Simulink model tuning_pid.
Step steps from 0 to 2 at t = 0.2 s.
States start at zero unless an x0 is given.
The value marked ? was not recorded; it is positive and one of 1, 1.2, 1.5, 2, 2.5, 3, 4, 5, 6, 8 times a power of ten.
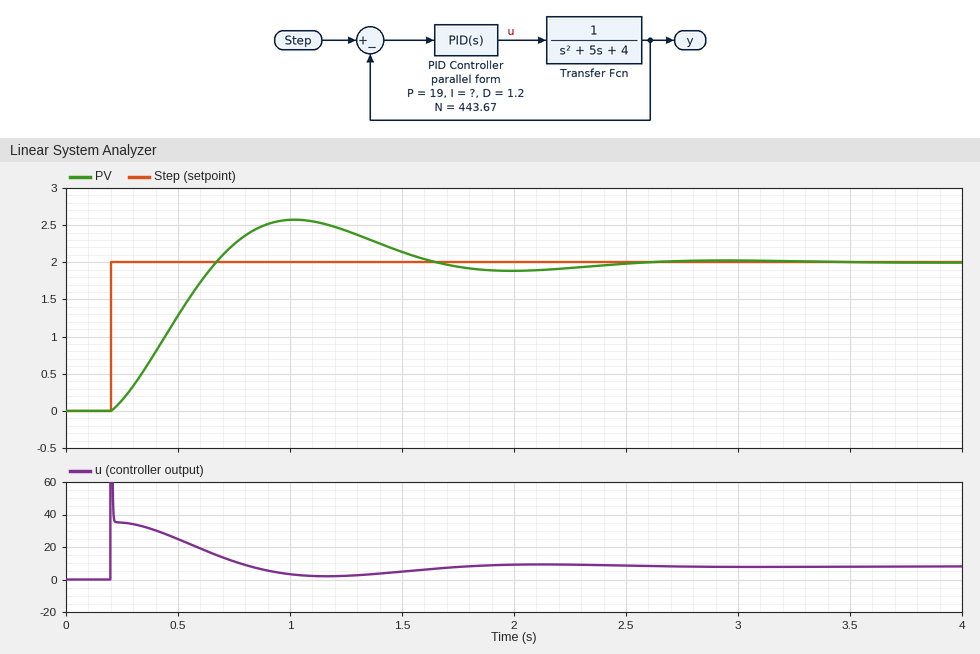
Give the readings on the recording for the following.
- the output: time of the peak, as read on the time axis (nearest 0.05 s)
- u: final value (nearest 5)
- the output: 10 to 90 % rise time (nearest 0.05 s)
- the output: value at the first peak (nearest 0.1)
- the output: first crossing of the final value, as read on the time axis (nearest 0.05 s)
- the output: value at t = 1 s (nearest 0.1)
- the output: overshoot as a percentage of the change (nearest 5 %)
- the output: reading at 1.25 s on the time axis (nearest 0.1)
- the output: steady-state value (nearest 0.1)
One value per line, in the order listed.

1.00 s
10
0.35 s
2.6
0.65 s
2.6
30 %
2.4
2.0
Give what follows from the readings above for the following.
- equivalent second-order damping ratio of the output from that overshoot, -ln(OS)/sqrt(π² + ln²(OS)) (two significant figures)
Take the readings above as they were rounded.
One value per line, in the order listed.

0.36
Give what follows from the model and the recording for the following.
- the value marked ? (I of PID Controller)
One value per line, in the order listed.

40
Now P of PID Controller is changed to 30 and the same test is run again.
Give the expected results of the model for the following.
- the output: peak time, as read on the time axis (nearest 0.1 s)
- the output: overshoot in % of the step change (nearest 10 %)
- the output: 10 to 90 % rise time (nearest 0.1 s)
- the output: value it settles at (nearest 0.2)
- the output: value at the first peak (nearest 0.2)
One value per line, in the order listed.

0.8 s
20 %
0.3 s
2.0
2.4
